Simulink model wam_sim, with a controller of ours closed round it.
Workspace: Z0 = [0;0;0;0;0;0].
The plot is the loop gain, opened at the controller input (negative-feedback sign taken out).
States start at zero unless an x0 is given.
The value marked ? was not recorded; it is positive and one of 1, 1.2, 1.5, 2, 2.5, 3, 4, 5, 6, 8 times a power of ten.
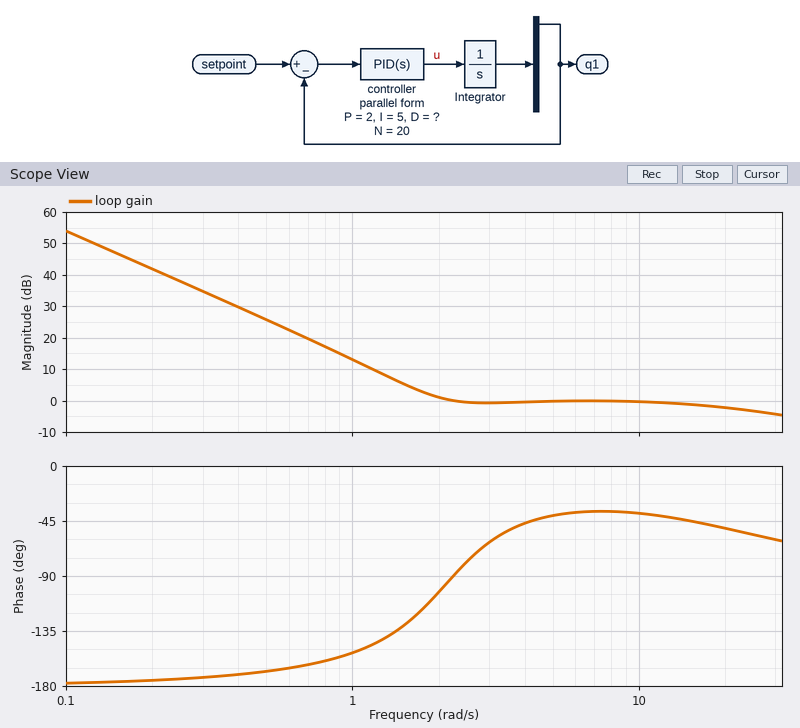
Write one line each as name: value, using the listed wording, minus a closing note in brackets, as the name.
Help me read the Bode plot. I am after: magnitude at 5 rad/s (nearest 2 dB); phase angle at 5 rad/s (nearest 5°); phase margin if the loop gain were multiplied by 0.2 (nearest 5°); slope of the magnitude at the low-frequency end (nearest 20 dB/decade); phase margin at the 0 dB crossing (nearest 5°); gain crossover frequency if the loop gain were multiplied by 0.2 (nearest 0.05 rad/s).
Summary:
magnitude at 5 rad/s: 0 dB
phase angle at 5 rad/s: -40°
phase margin if the loop gain were multiplied by 0.2: 25°
slope of the magnitude at the low-frequency end: -40 dB/decade
phase margin at the 0 dB crossing: 90°
gain crossover frequency if the loop gain were multiplied by 0.2: 0.95 rad/s
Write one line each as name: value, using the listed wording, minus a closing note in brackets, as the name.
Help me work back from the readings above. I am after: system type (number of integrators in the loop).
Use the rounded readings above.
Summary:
system type: 2
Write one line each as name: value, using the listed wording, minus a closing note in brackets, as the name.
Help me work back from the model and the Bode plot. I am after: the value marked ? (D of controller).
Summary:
the value marked ?: 1
